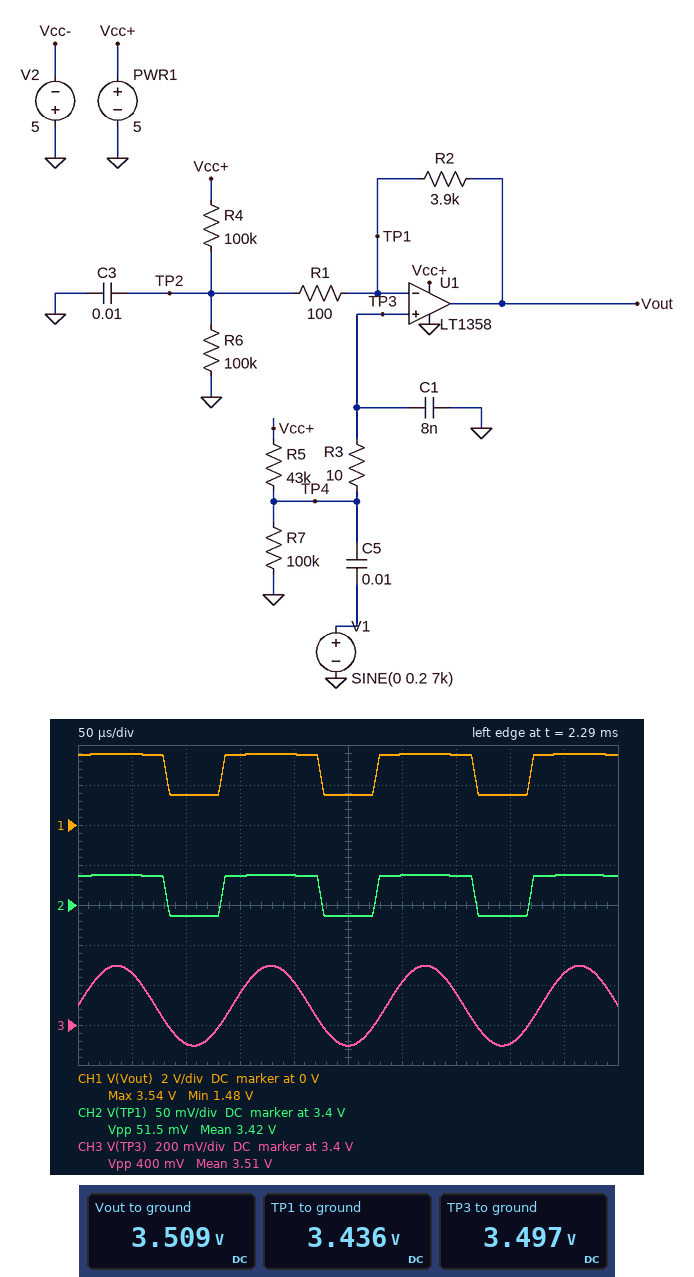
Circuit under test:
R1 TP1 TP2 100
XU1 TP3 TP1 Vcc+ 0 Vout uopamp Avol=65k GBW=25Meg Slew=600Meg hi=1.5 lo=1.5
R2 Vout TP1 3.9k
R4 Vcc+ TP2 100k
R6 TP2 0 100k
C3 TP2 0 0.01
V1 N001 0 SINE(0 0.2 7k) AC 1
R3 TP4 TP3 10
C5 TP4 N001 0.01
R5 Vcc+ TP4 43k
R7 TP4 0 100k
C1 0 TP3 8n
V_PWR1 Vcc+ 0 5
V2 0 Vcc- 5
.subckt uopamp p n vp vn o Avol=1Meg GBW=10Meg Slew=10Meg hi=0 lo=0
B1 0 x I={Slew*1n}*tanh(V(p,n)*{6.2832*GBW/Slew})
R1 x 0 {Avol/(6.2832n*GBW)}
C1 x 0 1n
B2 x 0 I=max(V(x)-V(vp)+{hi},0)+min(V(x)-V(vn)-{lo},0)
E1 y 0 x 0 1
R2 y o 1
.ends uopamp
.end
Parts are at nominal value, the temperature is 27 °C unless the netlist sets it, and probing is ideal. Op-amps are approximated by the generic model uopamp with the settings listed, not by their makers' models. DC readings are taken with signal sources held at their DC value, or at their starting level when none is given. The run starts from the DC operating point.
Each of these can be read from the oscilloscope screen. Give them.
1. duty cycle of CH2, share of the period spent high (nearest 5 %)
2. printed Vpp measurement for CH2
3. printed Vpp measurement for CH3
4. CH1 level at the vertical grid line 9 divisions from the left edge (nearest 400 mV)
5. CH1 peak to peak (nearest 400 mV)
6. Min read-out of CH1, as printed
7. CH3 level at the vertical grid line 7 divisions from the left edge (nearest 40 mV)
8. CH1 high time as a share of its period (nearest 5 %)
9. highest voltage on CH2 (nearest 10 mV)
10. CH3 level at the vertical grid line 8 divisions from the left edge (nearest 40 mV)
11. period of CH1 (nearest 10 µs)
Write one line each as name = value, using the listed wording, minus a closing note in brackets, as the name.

duty cycle of CH2, share of the period spent high = 65 %
printed Vpp measurement for CH2 = 51.5 mV
printed Vpp measurement for CH3 = 400 mV
CH1 level at the vertical grid line 9 divisions from the left edge = 3.6 V
CH1 peak to peak = 2.0 V
Min read-out of CH1, as printed = 1.48 V
CH3 level at the vertical grid line 7 divisions from the left edge = 3.56 V
CH1 high time as a share of its period = 65 %
highest voltage on CH2 = 3.44 V
CH3 level at the vertical grid line 8 divisions from the left edge = 3.32 V
period of CH1 = 140 µs
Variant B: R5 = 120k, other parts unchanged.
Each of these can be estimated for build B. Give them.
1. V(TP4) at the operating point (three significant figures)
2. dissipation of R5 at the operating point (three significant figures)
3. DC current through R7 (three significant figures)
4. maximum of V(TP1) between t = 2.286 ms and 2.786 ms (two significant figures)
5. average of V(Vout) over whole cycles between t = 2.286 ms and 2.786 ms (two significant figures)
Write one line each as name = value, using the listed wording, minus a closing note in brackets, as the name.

V(TP4) at the operating point = 2.27 V
dissipation of R5 at the operating point = 62.0 µW
DC current through R7 = 22.7 µA
maximum of V(TP1) between t = 2.286 ms and 2.786 ms = 2.3 V
average of V(Vout) over whole cycles between t = 2.286 ms and 2.786 ms = 2.5 V
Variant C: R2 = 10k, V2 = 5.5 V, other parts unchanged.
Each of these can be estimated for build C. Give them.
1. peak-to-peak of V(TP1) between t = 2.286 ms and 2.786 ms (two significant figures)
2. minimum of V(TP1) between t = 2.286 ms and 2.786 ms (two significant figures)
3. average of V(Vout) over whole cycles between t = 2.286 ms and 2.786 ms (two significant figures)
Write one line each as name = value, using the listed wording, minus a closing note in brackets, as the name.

peak-to-peak of V(TP1) between t = 2.286 ms and 2.786 ms = 20 mV
minimum of V(TP1) between t = 2.286 ms and 2.786 ms = 3.3 V
average of V(Vout) over whole cycles between t = 2.286 ms and 2.786 ms = 3.1 V
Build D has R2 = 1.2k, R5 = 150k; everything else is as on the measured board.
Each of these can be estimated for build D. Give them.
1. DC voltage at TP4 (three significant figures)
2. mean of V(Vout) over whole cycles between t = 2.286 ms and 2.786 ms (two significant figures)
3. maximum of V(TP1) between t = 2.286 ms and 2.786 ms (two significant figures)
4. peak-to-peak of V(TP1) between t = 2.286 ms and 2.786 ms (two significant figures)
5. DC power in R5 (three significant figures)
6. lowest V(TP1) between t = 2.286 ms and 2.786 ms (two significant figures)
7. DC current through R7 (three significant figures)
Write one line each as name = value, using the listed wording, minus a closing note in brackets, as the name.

DC voltage at TP4 = 2.00 V
mean of V(Vout) over whole cycles between t = 2.286 ms and 2.786 ms = 2.4 V
maximum of V(TP1) between t = 2.286 ms and 2.786 ms = 2.1 V
peak-to-peak of V(TP1) between t = 2.286 ms and 2.786 ms = 160 mV
DC power in R5 = 60.0 µW
lowest V(TP1) between t = 2.286 ms and 2.786 ms = 2.0 V
DC current through R7 = 20.0 µA
